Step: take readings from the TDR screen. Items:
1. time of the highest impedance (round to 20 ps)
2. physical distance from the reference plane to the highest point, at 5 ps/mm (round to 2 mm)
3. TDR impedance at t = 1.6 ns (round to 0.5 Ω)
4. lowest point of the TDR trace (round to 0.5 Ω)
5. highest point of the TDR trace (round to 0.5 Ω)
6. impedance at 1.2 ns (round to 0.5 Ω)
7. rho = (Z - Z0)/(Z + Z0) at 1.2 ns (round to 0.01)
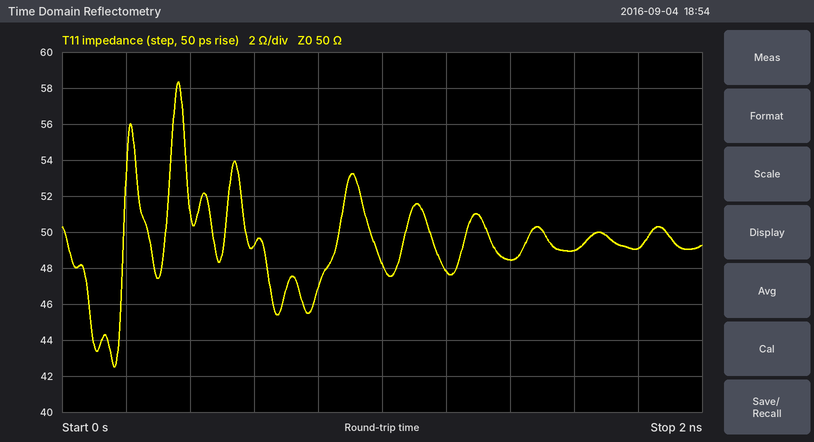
360 ps
36 mm
49.0 Ω
42.5 Ω
58.5 Ω
48.0 Ω
-0.02
